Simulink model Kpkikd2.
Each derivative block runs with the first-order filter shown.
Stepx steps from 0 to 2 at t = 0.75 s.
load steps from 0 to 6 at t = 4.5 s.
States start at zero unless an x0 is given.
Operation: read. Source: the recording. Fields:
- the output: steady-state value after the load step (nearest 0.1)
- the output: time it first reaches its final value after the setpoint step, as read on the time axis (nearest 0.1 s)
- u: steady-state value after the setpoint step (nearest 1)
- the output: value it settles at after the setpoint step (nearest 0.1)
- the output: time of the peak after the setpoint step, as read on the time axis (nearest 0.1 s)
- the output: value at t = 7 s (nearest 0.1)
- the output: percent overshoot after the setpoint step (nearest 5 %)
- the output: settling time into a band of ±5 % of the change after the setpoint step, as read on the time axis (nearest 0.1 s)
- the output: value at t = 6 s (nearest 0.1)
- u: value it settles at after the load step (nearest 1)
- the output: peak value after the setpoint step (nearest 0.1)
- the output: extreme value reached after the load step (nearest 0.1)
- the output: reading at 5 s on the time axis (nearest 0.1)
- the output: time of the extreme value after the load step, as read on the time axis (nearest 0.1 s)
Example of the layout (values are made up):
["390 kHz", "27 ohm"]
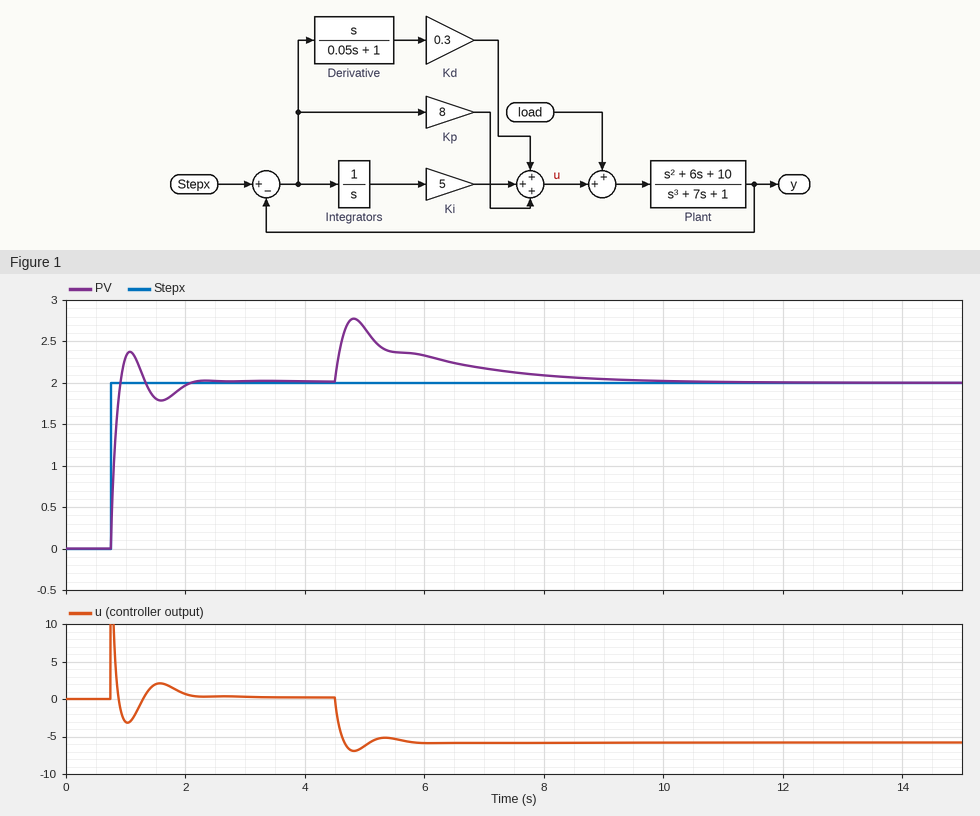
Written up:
["2.0", "0.9 s", "0", "2.0", "1.1 s", "2.2", "20 %", "1.9 s", "2.3", "-6", "2.4", "2.8", "2.7", "4.8 s"]
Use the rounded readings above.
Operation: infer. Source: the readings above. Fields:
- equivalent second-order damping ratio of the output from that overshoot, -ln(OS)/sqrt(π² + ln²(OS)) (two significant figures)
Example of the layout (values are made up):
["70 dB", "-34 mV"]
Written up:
["0.46"]
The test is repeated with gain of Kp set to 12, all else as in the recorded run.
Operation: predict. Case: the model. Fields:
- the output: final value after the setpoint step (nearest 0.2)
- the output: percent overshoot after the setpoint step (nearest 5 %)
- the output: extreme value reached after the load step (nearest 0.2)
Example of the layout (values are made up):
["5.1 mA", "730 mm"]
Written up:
["2.0", "15 %", "2.6"]
